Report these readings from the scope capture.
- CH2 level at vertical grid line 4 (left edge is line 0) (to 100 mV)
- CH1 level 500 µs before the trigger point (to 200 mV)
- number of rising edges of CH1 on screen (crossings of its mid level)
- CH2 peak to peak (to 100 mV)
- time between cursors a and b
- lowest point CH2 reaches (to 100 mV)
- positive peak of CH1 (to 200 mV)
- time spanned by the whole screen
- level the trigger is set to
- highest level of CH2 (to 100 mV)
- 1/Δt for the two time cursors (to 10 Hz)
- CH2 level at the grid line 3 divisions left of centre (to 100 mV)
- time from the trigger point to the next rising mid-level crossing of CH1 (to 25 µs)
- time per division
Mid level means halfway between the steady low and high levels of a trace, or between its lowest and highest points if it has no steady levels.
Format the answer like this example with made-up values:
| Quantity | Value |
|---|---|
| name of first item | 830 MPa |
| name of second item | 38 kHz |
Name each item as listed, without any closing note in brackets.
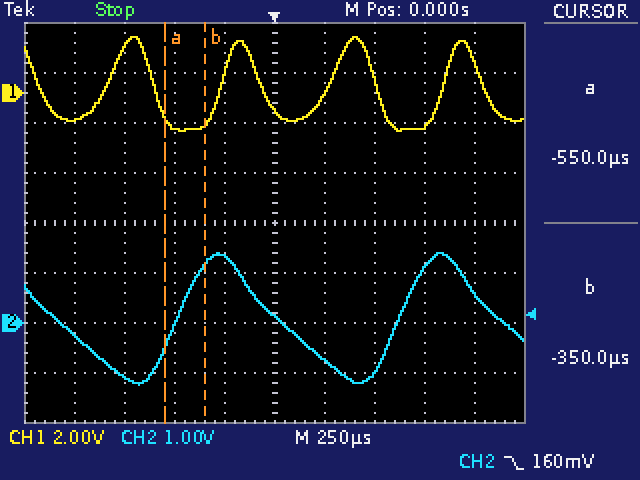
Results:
| Quantity | Value |
|---|---|
| CH2 level at vertical grid line 4 (left edge is line 0) | 1.3 V |
| CH1 level 500 µs before the trigger point | -1.4 V |
| number of rising edges of CH1 on screen | 4 |
| CH2 peak to peak | 2.6 V |
| time between cursors a and b | 200 µs |
| lowest point CH2 reaches | -1.2 V |
| positive peak of CH1 | 2.2 V |
| time spanned by the whole screen | 2.5 ms |
| level the trigger is set to | 160 mV |
| highest level of CH2 | 1.4 V |
| 1/Δt for the two time cursors | 5.00 kHz |
| CH2 level at the grid line 3 divisions left of centre | -1.1 V |
| time from the trigger point to the next rising mid-level crossing of CH1 | 275 µs |
| time per division | 250 µs |
